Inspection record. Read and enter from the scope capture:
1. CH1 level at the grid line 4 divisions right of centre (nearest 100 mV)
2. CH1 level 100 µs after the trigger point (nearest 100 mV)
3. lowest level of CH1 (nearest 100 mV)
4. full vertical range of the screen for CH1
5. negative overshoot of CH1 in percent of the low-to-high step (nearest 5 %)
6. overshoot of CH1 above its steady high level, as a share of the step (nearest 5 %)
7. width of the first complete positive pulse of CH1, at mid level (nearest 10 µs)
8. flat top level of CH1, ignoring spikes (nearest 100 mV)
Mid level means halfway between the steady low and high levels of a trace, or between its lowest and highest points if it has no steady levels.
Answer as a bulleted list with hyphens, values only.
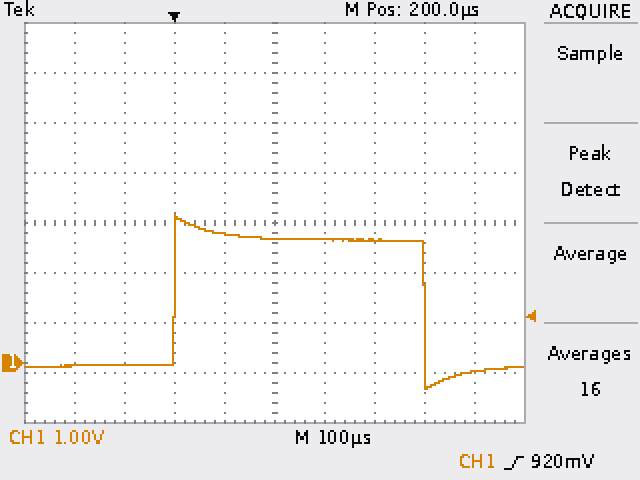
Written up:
- -200 mV
- 2.6 V
- -500 mV
- 8 V
- 20 %
- 20 %
- 500 µs
- 2.5 V
